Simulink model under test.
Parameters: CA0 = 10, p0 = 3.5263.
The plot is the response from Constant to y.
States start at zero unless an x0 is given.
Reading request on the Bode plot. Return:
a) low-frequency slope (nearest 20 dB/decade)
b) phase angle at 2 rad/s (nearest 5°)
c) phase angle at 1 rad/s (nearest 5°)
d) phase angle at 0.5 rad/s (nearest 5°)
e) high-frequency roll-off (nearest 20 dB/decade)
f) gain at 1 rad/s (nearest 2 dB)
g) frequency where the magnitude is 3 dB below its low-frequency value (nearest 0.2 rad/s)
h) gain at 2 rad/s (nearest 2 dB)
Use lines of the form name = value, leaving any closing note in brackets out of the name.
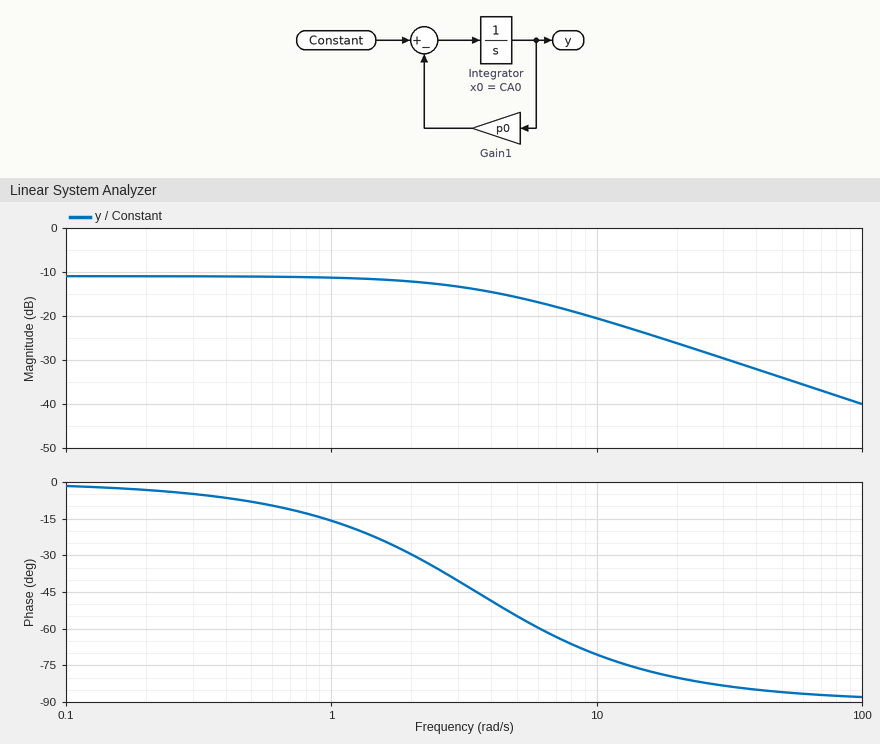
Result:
low-frequency slope = 0 dB/decade
phase angle at 2 rad/s = -30°
phase angle at 1 rad/s = -15°
phase angle at 0.5 rad/s = -10°
high-frequency roll-off = -20 dB/decade
gain at 1 rad/s = -12 dB
frequency where the magnitude is 3 dB below its low-frequency value = 3.6 rad/s
gain at 2 rad/s = -12 dB
